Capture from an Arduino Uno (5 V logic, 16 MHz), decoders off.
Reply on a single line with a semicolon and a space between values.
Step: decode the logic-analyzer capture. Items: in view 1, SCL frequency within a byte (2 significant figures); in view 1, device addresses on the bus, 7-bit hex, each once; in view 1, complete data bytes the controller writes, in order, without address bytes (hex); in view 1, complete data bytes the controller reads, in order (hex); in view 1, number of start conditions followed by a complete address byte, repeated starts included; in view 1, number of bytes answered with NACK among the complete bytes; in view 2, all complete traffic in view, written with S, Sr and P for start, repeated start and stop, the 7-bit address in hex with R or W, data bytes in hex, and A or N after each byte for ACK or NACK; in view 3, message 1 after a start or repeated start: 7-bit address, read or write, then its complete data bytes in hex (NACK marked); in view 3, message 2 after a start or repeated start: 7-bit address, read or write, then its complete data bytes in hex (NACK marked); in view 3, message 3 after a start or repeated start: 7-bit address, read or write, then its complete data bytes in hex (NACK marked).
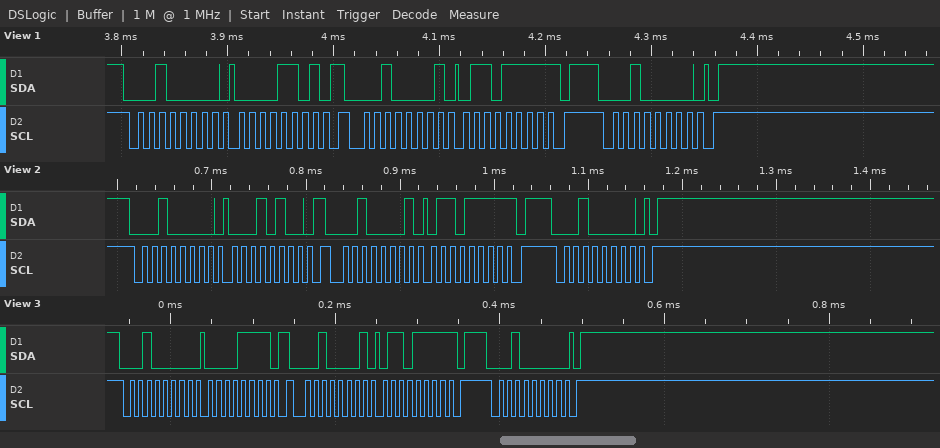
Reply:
100 kHz; 0x10; 0D; 6F; 3; 1; S 10W A 14 A Sr 10R A 6F N P S 10W A P; 0x10 write: 0F; 0x10 read: 6F NACK; 0x10 write
